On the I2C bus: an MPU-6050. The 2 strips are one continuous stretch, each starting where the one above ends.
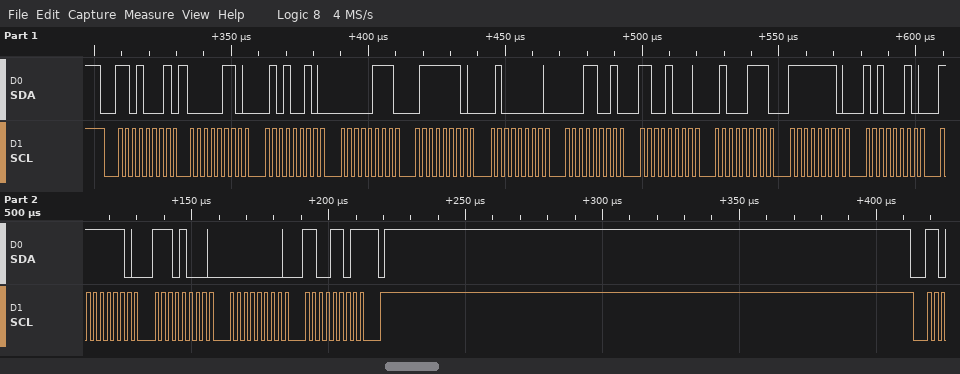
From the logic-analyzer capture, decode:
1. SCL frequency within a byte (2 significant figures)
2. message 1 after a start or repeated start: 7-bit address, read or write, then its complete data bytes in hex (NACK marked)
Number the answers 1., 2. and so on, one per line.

1. 400 kHz
2. 0x68 read: 06 52 07 7E 40 19 C8 47 FE A2 FE E8 00 CD NACK
